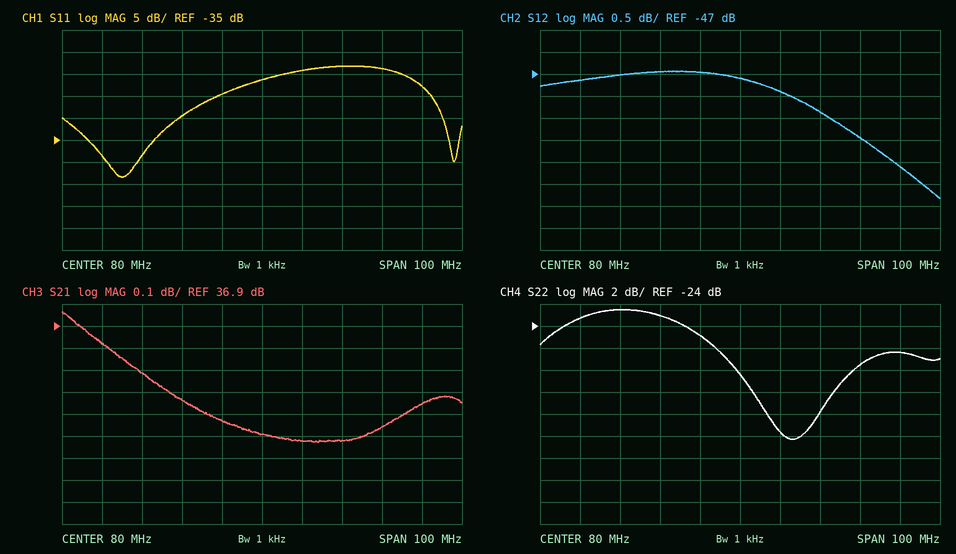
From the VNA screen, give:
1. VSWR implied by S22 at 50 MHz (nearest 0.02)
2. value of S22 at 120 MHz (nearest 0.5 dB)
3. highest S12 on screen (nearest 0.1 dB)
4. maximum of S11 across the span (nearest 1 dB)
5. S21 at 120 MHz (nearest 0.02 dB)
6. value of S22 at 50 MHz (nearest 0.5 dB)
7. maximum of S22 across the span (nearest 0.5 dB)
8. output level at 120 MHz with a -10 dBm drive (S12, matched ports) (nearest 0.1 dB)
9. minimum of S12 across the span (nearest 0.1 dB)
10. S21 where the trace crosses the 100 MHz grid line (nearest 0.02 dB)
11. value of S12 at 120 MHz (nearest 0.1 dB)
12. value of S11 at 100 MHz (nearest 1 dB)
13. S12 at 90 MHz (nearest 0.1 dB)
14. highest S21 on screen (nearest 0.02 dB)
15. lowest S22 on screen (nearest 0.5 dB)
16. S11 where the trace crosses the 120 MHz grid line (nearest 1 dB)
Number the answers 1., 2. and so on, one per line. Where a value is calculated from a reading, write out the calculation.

1. |Γ| = 10^(-22.5/20) = 0.0750; VSWR = (1 + 0.0750)/(1 − 0.0750) ≈ 1.16
2. -26.5 dB
3. -46.9 dB
4. -18 dB
5. 36.54 dB
6. -22.5 dB
7. -22.5 dB
8. -10 dBm + (-49.1 dB) = -59.1 dBm
9. -49.8 dB
10. 36.38 dB
11. -49.1 dB
12. -18 dB
13. -47.4 dB
14. 36.96 dB
15. -34.5 dB
16. -23 dB
